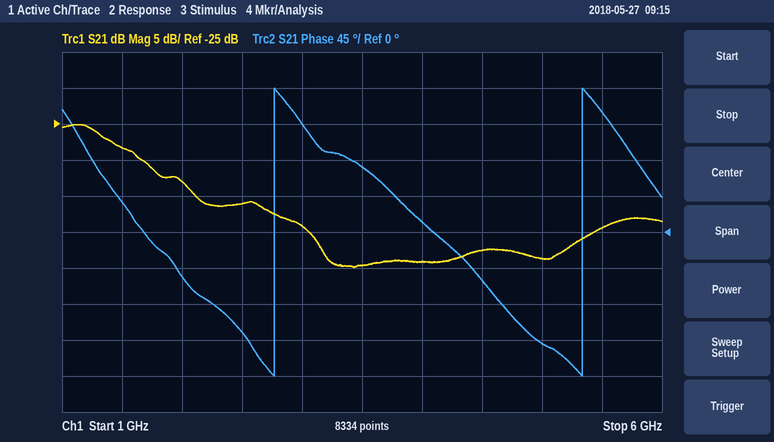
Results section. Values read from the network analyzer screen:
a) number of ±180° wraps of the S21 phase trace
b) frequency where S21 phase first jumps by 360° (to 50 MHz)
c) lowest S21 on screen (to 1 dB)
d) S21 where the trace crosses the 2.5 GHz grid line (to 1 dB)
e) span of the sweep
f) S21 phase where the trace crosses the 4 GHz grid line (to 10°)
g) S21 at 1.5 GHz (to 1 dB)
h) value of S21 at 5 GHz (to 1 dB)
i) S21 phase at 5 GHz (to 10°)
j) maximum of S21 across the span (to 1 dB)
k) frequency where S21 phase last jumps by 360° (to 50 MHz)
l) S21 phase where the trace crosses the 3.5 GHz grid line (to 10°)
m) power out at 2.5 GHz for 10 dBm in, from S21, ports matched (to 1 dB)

2
2.75 GHz
-45 dB
-36 dB
5 GHz
10°
-28 dB
-44 dB
-140°
-25 dB
5.35 GHz
80°
-26 dBm
